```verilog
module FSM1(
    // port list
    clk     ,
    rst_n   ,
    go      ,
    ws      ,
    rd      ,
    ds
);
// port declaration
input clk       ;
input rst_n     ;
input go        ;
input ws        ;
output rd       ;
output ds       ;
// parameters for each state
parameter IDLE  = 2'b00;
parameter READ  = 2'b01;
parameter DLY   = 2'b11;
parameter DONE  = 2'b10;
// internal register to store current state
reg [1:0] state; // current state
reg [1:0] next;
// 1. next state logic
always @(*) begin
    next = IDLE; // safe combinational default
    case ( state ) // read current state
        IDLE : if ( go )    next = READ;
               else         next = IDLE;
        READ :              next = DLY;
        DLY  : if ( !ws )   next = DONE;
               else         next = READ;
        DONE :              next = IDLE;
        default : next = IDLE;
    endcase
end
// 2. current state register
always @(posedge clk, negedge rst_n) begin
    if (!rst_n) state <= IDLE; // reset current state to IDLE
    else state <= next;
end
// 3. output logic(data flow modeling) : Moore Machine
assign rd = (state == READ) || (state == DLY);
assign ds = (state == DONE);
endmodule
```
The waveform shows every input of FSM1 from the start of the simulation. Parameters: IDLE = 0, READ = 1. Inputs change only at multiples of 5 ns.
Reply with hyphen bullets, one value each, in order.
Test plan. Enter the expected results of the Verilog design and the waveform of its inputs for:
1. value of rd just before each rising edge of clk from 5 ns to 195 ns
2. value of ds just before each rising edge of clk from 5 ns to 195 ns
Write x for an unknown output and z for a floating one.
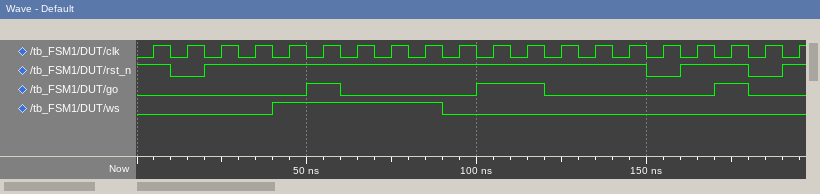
- x 0 0 0 0 0 1 1 1 1 0 0 1 1 0 0 0 0 0 0
- x 0 0 0 0 0 0 0 0 0 1 0 0 0 1 0 0 0 0 0
